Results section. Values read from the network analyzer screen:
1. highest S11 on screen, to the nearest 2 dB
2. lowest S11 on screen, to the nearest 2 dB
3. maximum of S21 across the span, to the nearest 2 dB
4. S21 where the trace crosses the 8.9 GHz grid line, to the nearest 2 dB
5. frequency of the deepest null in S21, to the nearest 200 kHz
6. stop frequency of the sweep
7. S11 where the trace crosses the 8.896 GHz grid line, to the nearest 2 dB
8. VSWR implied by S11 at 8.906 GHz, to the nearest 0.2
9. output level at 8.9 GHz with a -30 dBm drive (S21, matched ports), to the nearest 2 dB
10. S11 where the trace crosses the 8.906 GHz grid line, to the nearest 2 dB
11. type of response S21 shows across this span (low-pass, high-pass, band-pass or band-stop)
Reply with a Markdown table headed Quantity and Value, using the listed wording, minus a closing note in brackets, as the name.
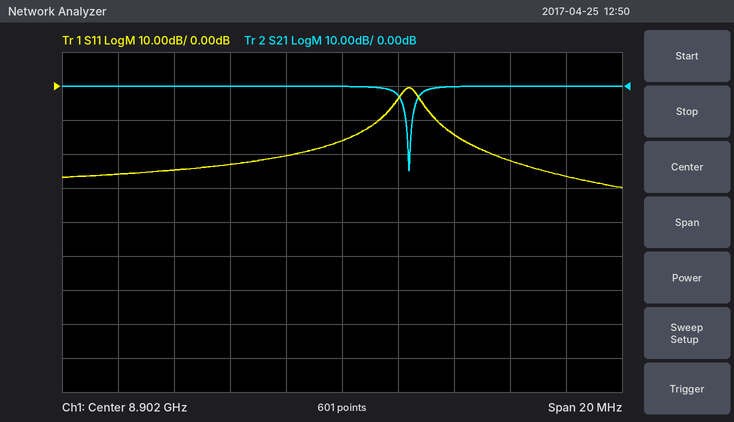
| Quantity | Value |
|---|---|
| highest S11 on screen, to the nearest 2 dB | 0 dB |
| lowest S11 on screen, to the nearest 2 dB | -30 dB |
| maximum of S21 across the span, to the nearest 2 dB | 0 dB |
| S21 where the trace crosses the 8.9 GHz grid line, to the nearest 2 dB | 0 dB |
| frequency of the deepest null in S21, to the nearest 200 kHz | 8.9044 GHz |
| stop frequency of the sweep | 8.912 GHz |
| S11 where the trace crosses the 8.896 GHz grid line, to the nearest 2 dB | -24 dB |
| VSWR implied by S11 at 8.906 GHz, to the nearest 0.2 | 1.4 |
| output level at 8.9 GHz with a -30 dBm drive (S21, matched ports), to the nearest 2 dB | -30 dBm |
| S11 where the trace crosses the 8.906 GHz grid line, to the nearest 2 dB | -14 dB |
| type of response S21 shows across this span | band-stop |
